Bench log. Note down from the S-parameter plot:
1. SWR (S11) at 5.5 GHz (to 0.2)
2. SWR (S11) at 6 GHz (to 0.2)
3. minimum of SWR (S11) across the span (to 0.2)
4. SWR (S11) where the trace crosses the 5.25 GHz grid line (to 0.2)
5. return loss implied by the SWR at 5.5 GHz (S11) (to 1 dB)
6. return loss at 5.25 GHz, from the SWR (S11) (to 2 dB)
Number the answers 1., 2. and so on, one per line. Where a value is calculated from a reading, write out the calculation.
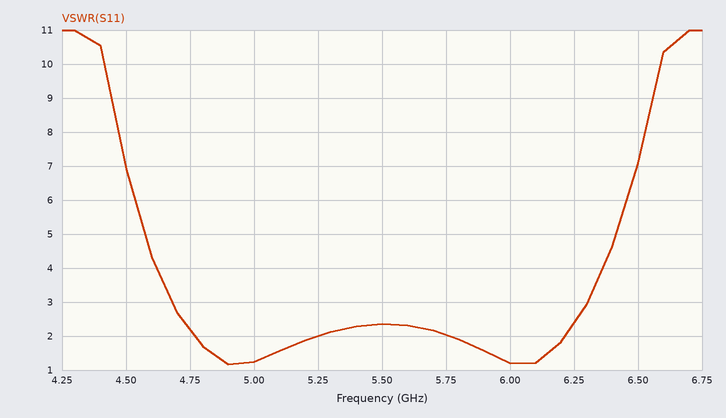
1. 2.4
2. 1.2
3. 1.2
4. 2.0
5. −20 log10((2.4 − 1)/(2.4 + 1)) ≈ 8 dB
6. −20 log10((2 − 1)/(2 + 1)) ≈ 10 dB
